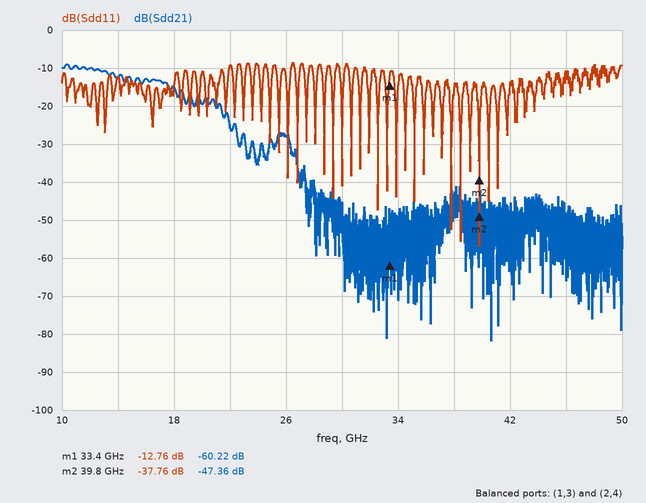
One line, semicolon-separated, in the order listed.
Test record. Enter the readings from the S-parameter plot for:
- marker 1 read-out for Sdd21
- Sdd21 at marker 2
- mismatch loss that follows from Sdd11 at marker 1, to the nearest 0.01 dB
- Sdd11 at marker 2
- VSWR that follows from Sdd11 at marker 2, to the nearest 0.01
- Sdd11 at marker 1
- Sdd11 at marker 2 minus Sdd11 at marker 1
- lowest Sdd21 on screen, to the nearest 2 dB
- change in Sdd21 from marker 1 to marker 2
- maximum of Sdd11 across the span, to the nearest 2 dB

-60.22 dB; -47.36 dB; 0.24 dB; -37.76 dB; 1.03; -12.76 dB; -25.00 dB; -82 dB; 12.86 dB; -8 dB
